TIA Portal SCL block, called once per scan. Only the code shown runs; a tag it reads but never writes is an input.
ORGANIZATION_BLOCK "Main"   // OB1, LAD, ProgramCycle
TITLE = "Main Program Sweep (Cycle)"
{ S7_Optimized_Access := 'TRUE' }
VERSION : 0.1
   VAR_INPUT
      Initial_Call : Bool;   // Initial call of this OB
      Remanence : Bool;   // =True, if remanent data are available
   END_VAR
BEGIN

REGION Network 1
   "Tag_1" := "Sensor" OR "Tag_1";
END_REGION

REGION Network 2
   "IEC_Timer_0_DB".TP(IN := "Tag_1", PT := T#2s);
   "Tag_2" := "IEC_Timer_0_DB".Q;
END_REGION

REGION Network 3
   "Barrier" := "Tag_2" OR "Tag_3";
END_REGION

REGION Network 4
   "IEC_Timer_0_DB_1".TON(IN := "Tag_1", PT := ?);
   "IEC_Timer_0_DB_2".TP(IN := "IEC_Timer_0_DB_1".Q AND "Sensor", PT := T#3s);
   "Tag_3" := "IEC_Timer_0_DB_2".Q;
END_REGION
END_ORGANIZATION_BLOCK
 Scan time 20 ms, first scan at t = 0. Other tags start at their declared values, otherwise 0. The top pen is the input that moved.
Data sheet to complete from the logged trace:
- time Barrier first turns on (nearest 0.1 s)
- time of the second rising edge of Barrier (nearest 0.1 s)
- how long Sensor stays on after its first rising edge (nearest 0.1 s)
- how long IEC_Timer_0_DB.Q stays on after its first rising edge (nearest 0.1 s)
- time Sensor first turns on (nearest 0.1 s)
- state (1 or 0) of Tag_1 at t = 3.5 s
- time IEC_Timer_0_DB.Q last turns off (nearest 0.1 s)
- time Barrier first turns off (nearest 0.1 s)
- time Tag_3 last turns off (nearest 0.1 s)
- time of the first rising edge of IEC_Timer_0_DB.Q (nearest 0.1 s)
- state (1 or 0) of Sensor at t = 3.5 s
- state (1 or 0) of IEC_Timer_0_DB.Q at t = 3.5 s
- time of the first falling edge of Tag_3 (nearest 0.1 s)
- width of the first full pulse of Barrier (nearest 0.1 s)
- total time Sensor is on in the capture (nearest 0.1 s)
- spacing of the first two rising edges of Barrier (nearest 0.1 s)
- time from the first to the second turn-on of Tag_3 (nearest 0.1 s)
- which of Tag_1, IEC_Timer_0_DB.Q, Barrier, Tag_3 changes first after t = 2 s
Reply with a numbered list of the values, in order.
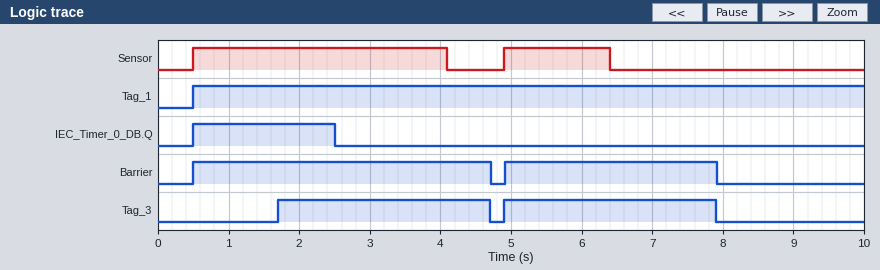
1. 0.5 s
2. 4.9 s
3. 3.6 s
4. 2.0 s
5. 0.5 s
6. 1
7. 2.5 s
8. 4.7 s
9. 7.9 s
10. 0.5 s
11. 1
12. 0
13. 4.7 s
14. 4.2 s
15. 5.1 s
16. 4.4 s
17. 3.2 s
18. IEC_Timer_0_DB.Q
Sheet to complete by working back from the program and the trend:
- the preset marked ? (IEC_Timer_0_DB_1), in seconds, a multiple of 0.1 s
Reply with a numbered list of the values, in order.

1. 1.2 s
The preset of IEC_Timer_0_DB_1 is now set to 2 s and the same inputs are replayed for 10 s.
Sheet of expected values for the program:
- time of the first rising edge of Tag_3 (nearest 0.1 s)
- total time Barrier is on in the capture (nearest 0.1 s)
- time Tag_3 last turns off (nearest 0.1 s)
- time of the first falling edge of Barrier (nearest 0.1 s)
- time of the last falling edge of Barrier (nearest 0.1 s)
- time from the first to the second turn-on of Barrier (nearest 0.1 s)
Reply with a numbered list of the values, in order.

1. 2.5 s
2. 5.0 s
3. 5.5 s
4. 2.5 s
5. 5.5 s
6. 2.0 s
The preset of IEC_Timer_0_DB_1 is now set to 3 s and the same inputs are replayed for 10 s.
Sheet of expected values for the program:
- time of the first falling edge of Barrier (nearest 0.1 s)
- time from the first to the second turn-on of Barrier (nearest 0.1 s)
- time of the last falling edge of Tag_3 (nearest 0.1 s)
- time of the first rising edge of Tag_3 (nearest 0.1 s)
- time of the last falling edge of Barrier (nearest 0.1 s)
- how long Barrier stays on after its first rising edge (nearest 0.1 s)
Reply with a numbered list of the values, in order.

1. 2.5 s
2. 3.0 s
3. 6.5 s
4. 3.5 s
5. 6.5 s
6. 2.0 s
